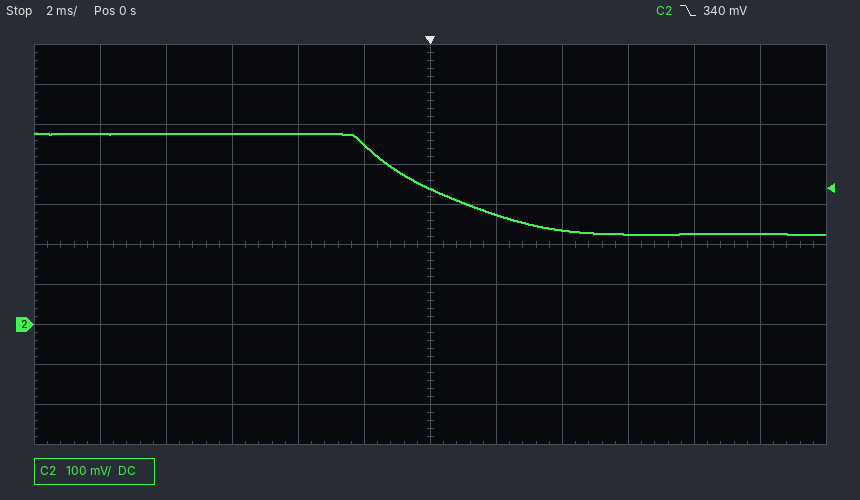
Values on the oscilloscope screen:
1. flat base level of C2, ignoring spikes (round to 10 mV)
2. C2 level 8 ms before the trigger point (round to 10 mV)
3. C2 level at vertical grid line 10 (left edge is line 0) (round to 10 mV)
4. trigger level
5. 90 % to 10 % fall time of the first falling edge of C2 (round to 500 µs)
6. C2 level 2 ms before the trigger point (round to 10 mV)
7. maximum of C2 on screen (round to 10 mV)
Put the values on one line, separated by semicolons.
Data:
230 mV; 480 mV; 230 mV; 340 mV; 5.0 ms; 450 mV; 480 mV
